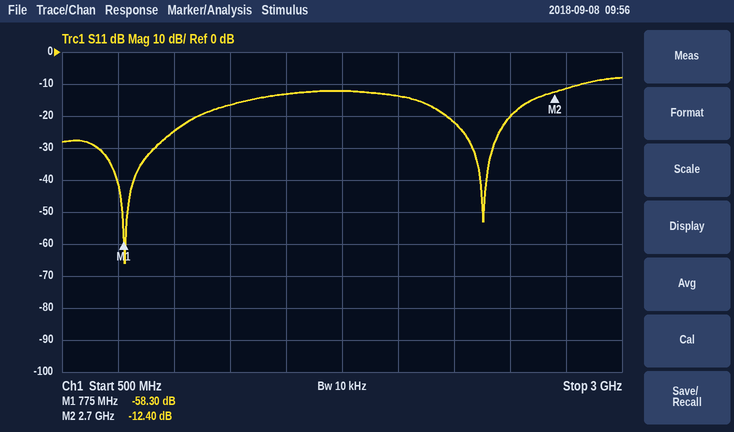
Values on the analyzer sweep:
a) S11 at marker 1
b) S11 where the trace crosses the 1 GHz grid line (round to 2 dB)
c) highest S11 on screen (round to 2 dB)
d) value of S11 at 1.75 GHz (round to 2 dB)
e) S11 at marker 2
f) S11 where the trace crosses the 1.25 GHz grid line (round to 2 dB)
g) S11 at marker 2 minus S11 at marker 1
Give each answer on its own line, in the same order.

-58.30 dB
-24 dB
-8 dB
-12 dB
-12.40 dB
-16 dB
45.90 dB
